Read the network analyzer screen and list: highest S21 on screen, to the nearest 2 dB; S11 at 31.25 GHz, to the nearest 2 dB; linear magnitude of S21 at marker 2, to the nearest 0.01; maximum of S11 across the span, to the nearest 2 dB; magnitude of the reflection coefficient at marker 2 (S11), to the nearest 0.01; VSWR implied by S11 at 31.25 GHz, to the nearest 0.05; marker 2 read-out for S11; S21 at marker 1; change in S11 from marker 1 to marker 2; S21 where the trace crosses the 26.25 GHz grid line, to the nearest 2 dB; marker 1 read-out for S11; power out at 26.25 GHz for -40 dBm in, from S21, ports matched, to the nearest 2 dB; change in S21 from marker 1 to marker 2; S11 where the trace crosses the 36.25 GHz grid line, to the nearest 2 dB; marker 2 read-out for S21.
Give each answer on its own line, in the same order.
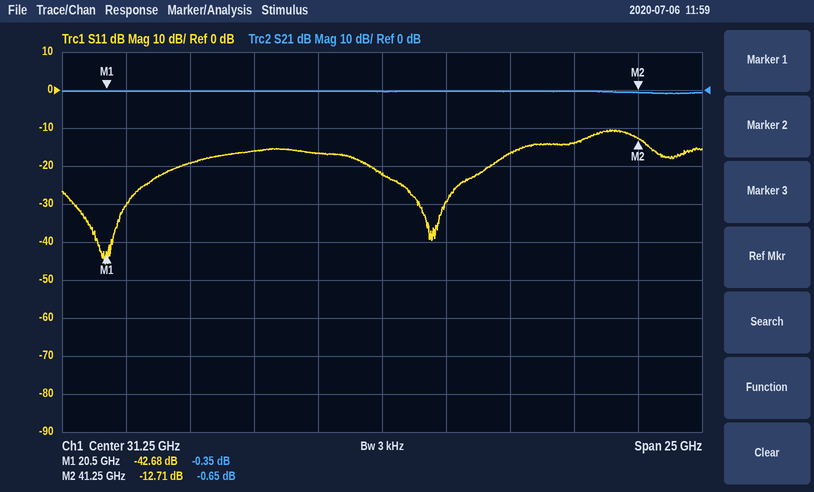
0 dB
-22 dB
0.93
-10 dB
0.23
1.15
-12.71 dB
-0.35 dB
29.97 dB
0 dB
-42.68 dB
-40 dBm
-0.30 dB
-16 dB
-0.65 dB
